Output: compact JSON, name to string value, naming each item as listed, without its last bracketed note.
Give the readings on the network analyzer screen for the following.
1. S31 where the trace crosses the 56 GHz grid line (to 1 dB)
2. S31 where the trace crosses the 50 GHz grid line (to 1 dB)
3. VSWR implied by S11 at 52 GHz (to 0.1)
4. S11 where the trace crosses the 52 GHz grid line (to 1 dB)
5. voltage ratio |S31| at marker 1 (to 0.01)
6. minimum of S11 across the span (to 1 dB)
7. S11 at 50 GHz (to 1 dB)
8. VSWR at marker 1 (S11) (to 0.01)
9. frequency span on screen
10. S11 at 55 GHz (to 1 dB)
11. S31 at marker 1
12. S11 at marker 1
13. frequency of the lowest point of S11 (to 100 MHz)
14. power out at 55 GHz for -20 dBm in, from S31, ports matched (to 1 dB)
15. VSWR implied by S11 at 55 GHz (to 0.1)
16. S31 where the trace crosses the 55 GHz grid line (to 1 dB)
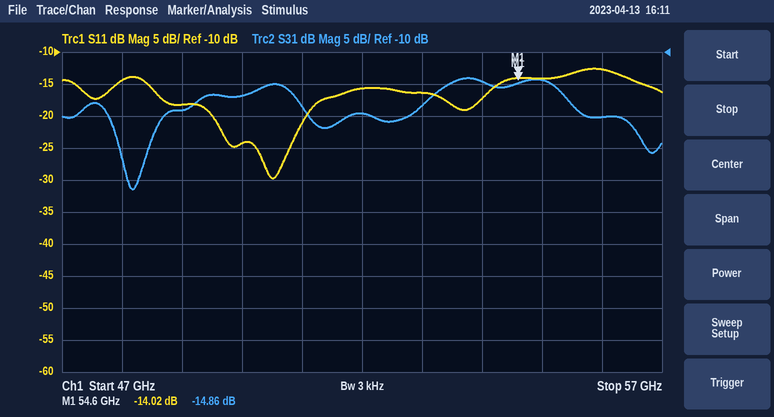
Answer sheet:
{"S31 where the trace crosses the 56 GHz grid line": "-20 dB", "S31 where the trace crosses the 50 GHz grid line": "-17 dB", "VSWR implied by S11 at 52 GHz": "1.4", "S11 where the trace crosses the 52 GHz grid line": "-16 dB", "voltage ratio |S31| at marker 1": "0.18", "minimum of S11 across the span": "-30 dB", "S11 at 50 GHz": "-24 dB", "VSWR at marker 1 (S11)": "1.50", "frequency span on screen": "10 GHz", "S11 at 55 GHz": "-14 dB", "S31 at marker 1": "-14.86 dB", "S11 at marker 1": "-14.02 dB", "frequency of the lowest point of S11": "50.5 GHz", "power out at 55 GHz for -20 dBm in, from S31, ports matched": "-34 dBm", "VSWR implied by S11 at 55 GHz": "1.5", "S31 where the trace crosses the 55 GHz grid line": "-14 dB"}
